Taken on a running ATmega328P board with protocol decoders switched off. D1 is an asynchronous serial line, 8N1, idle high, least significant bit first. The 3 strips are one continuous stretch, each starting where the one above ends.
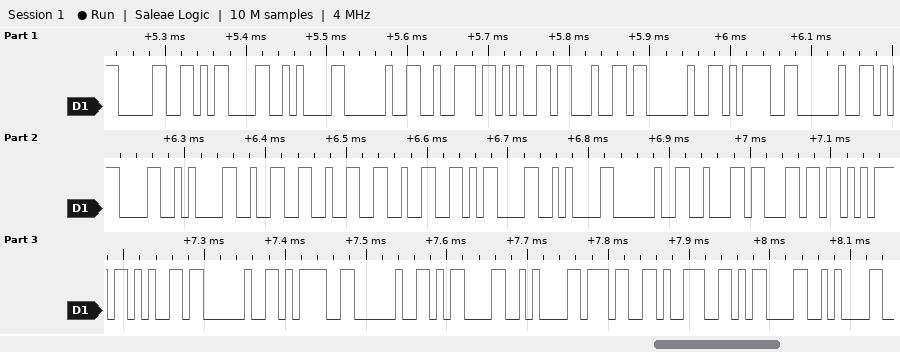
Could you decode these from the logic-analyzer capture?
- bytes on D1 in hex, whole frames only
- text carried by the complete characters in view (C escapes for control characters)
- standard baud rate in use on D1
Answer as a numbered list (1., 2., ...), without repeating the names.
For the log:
1. 30 0D 0A 20 72 65 64 20 3D 20 0D 0A 32 32 32 0D 0A 20 62 6C 75 65 20 3D 20 0D 0A 37 39 0D 0A
2. "0\r\n red = \r\n222\r\n blue = \r\n79\r\n"
3. 115200 baud
